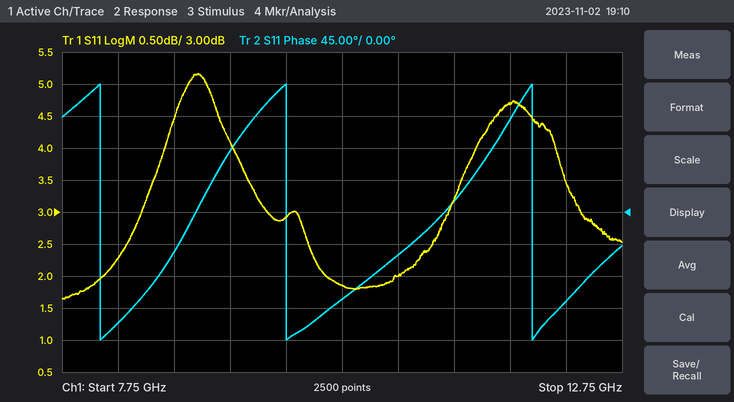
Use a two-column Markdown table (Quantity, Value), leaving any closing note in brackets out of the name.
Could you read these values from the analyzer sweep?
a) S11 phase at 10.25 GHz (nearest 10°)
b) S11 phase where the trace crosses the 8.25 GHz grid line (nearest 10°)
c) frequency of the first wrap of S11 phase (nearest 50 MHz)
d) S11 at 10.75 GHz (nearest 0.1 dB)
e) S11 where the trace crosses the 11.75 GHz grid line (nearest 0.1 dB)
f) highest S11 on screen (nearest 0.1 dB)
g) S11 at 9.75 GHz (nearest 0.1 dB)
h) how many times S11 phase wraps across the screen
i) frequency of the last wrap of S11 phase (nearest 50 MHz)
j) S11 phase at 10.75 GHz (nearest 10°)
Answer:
| Quantity | Value |
|---|---|
| S11 phase at 10.25 GHz | -120° |
| S11 phase where the trace crosses the 8.25 GHz grid line | -160° |
| frequency of the first wrap of S11 phase | 8.10 GHz |
| S11 at 10.75 GHz | 2.0 dB |
| S11 where the trace crosses the 11.75 GHz grid line | 4.7 dB |
| highest S11 on screen | 5.2 dB |
| S11 at 9.75 GHz | 2.9 dB |
| how many times S11 phase wraps across the screen | 3 |
| frequency of the last wrap of S11 phase | 11.95 GHz |
| S11 phase at 10.75 GHz | -60° |
